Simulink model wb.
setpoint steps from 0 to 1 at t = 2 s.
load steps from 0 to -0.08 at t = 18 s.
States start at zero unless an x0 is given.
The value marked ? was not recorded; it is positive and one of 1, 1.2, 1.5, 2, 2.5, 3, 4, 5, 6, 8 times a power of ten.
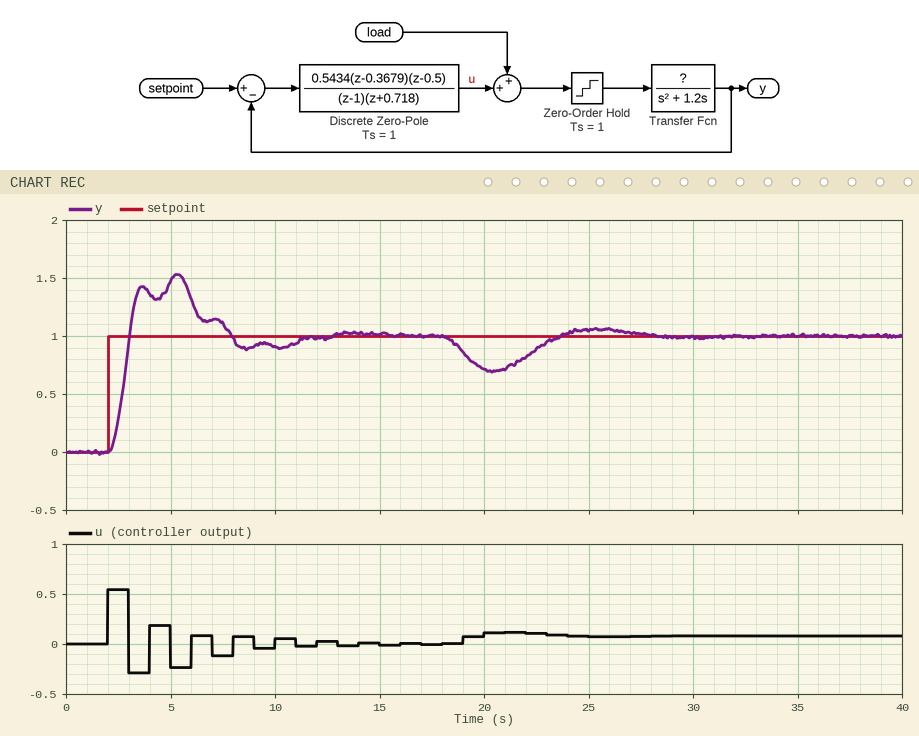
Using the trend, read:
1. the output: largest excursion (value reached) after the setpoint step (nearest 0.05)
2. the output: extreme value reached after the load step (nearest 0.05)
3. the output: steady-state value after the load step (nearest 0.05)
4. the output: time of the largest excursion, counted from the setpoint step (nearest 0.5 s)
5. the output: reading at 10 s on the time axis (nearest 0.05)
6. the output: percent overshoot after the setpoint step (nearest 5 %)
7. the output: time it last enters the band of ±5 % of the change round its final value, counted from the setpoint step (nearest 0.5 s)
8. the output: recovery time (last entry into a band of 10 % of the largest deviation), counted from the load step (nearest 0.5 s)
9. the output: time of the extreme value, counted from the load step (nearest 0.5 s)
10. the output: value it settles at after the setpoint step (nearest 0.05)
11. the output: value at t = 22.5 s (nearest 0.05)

1.55
0.70
1.00
3.5 s
0.90
55 %
9.0 s
9.0 s
2.5 s
1.00
0.90
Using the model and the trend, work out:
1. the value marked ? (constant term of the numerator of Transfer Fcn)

5
